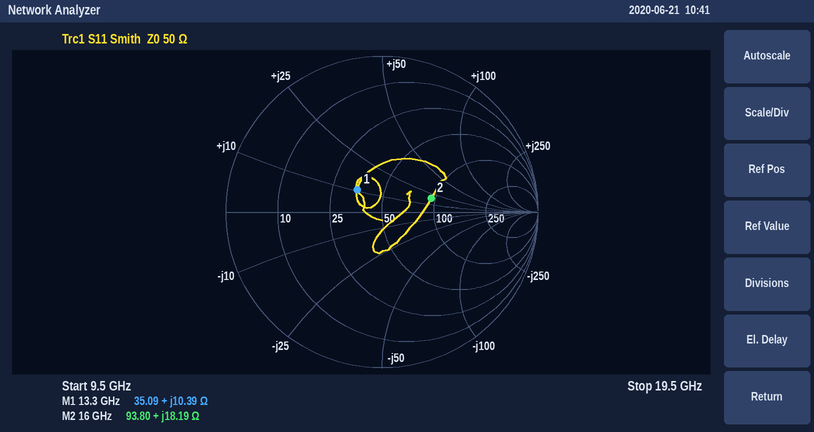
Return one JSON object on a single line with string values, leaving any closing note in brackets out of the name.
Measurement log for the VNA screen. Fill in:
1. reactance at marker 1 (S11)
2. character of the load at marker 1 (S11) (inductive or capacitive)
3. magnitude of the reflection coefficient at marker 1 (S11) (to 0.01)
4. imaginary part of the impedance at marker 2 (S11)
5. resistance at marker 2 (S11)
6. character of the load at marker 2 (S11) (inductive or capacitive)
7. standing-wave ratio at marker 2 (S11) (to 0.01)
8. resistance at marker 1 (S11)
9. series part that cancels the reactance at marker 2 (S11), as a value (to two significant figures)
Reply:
{"reactance at marker 1": "+10.39 Ω", "character of the load at marker 1 (S11)": "inductive", "magnitude of the reflection coefficient at marker 1 (S11)": "0.21", "imaginary part of the impedance at marker 2": "+18.19 Ω", "resistance at marker 2": "93.80 Ω", "character of the load at marker 2 (S11)": "inductive", "standing-wave ratio at marker 2 (S11)": "1.97", "resistance at marker 1": "35.09 Ω", "series part that cancels the reactance at marker 2 (S11), as a value": "550 fF"}
